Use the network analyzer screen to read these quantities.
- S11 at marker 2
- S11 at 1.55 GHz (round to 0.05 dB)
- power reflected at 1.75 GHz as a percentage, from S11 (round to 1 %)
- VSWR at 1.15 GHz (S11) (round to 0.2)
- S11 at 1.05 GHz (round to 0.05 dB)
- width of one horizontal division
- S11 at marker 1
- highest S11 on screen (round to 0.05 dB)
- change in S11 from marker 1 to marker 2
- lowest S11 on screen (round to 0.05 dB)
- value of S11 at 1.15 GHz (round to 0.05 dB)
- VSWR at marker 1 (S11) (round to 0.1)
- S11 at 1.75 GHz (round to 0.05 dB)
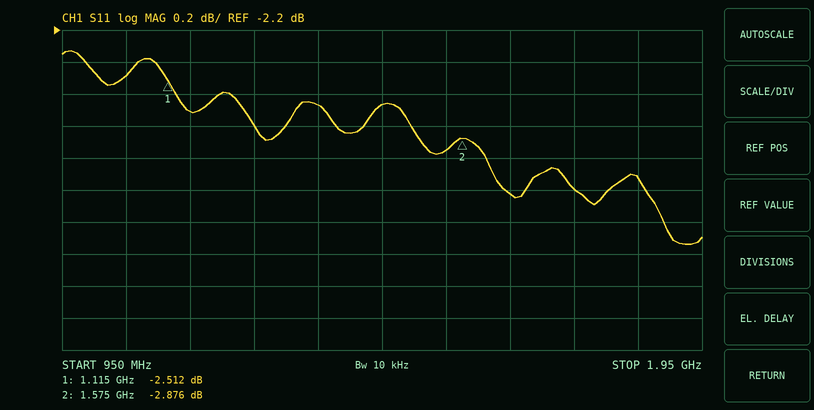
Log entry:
-2.876 dB
-2.95 dB
48 %
6.4
-2.50 dB
100 MHz
-2.512 dB
-2.35 dB
-0.364 dB
-3.55 dB
-2.70 dB
7.0
-3.20 dB
